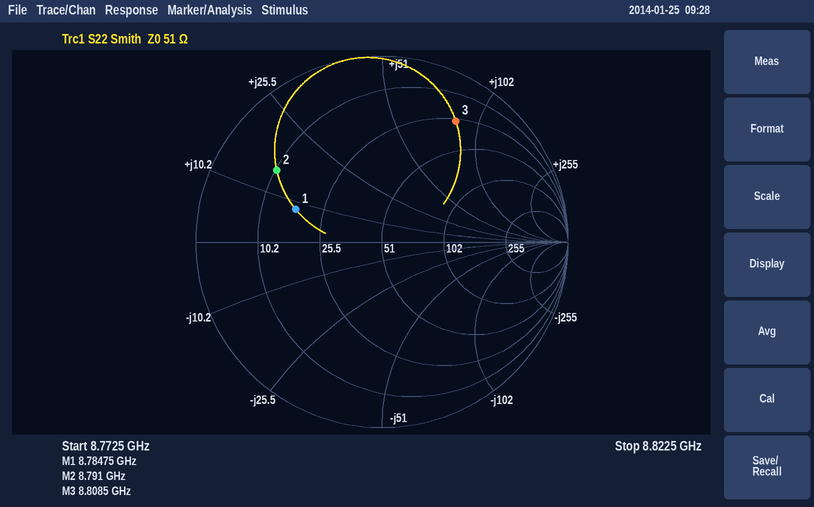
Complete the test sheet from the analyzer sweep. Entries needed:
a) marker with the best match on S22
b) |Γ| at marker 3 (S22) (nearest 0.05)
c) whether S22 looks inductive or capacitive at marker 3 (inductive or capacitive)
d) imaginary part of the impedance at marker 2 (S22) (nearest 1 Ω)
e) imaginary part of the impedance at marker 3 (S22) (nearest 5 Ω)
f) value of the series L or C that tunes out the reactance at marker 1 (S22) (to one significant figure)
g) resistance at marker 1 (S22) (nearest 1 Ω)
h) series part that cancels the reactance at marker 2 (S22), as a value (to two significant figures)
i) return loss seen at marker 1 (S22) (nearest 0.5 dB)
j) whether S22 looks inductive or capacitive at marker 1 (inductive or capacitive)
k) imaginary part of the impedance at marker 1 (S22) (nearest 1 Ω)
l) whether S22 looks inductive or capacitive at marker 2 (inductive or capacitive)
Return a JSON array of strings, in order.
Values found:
["marker 1", "0.75", "inductive", "+15 Ω", "+85 Ω", "2 pF", "18 Ω", "1.2 pF", "6.0 dB", "inductive", "+8 Ω", "inductive"]
